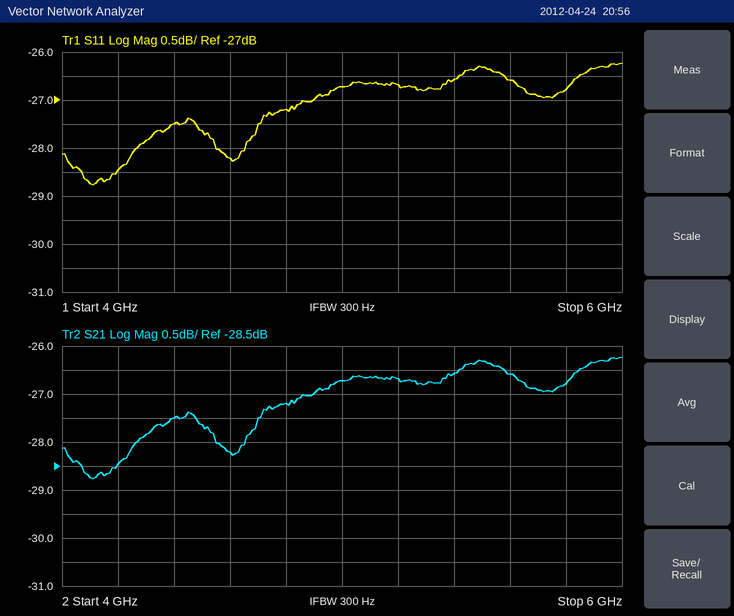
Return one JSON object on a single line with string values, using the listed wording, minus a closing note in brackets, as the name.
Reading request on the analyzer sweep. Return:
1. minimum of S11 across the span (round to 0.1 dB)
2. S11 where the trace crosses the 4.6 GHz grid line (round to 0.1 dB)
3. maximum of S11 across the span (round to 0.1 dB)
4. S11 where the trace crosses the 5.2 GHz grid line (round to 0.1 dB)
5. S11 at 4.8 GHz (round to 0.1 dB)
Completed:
{"minimum of S11 across the span": "-28.8 dB", "S11 where the trace crosses the 4.6 GHz grid line": "-28.2 dB", "maximum of S11 across the span": "-26.2 dB", "S11 where the trace crosses the 5.2 GHz grid line": "-26.7 dB", "S11 at 4.8 GHz": "-27.2 dB"}
